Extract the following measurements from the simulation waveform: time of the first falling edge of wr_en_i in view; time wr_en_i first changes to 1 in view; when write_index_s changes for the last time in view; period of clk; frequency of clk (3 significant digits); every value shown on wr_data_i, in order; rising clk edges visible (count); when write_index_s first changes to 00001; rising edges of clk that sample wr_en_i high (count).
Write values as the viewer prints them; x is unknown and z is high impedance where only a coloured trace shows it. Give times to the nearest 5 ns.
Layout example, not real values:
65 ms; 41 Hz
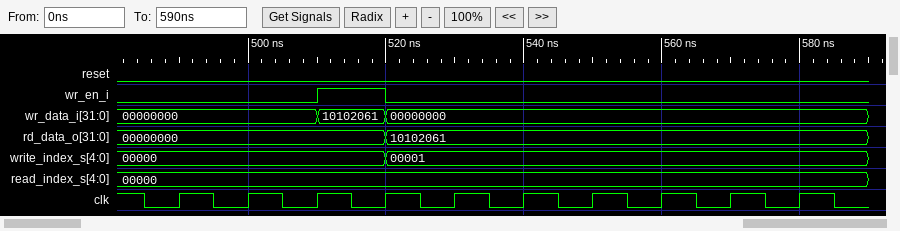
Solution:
520 ns; 510 ns; 520 ns; 10 ns; 100 MHz; 00000000, 10102061, 00000000; 10; 520 ns; 1
